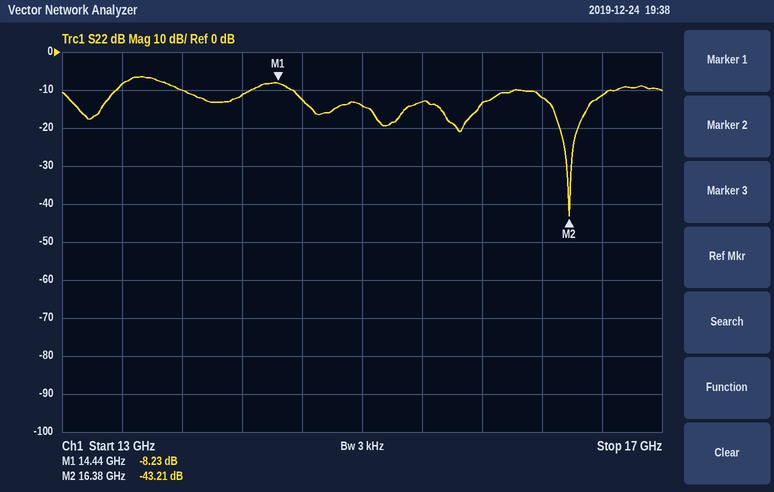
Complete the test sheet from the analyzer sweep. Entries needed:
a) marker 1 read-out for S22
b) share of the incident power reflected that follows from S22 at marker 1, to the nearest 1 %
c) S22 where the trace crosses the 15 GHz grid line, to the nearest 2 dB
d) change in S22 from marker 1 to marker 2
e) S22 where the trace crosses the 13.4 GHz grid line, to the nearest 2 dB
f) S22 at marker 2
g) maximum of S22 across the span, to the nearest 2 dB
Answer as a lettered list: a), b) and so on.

a) -8.23 dB
b) 15 %
c) -14 dB
d) -34.98 dB
e) -8 dB
f) -43.21 dB
g) -6 dB
